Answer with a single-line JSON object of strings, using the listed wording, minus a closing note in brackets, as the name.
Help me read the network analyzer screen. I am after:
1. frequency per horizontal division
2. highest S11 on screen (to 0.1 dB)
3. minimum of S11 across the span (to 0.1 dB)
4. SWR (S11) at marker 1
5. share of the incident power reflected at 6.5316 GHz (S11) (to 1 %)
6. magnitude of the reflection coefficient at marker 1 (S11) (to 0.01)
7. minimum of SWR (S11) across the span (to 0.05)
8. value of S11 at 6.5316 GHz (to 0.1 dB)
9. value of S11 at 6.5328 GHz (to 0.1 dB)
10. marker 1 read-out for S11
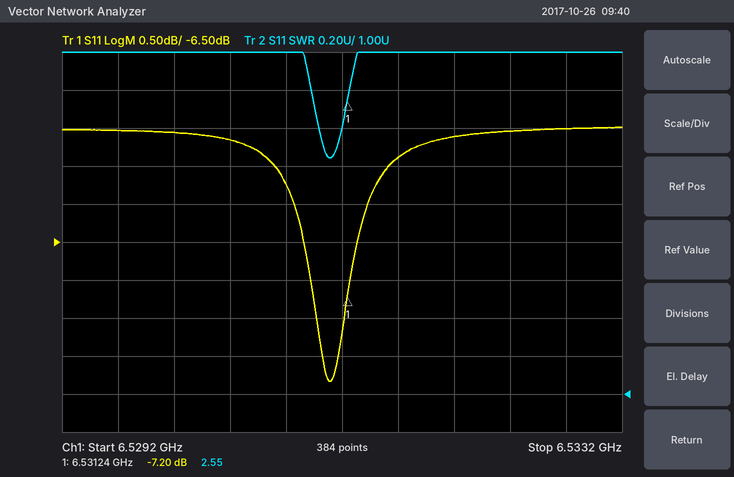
{"frequency per horizontal division": "400 kHz", "highest S11 on screen": "-5.0 dB", "minimum of S11 across the span": "-8.3 dB", "SWR (S11) at marker 1": "2.55", "share of the incident power reflected at 6.5316 GHz (S11)": "29 %", "magnitude of the reflection coefficient at marker 1 (S11)": "0.44", "minimum of SWR (S11) across the span": "2.25", "value of S11 at 6.5316 GHz": "-5.4 dB", "value of S11 at 6.5328 GHz": "-5.0 dB", "marker 1 read-out for S11": "-7.20 dB"}
